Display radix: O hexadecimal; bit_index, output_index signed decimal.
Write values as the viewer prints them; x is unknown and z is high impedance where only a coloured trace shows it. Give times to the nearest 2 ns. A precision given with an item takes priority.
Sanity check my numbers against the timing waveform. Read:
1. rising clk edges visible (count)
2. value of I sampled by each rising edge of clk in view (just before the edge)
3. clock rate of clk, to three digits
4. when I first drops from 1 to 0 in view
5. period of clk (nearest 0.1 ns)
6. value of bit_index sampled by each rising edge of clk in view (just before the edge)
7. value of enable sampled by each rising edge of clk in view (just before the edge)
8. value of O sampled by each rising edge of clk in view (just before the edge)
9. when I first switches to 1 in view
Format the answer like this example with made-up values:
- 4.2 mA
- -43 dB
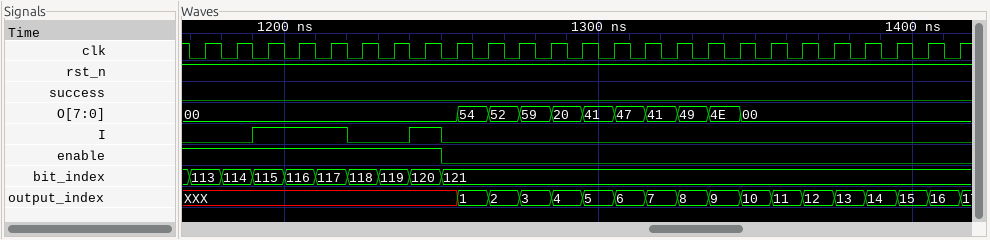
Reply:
- 25
- 0 0 1 1 1 0 0 1 0 0 0 0 0 0 0 0 0 0 0 0 0 0 0 0 0
- 100 MHz
- 1220 ns
- 10 ns
- 113, 114, 115, 116, 117, 118, 119, 120, 121, 121, 121, 121, 121, 121, 121, 121, 121, 121, 121, 121, 121, 121, 121, 121, 121
- 1 1 1 1 1 1 1 1 0 0 0 0 0 0 0 0 0 0 0 0 0 0 0 0 0
- 00, 00, 00, 00, 00, 00, 00, 00, 00, 54, 52, 59, 20, 41, 47, 41, 49, 4E, 00, 00, 00, 00, 00, 00, 00
- 1190 ns
